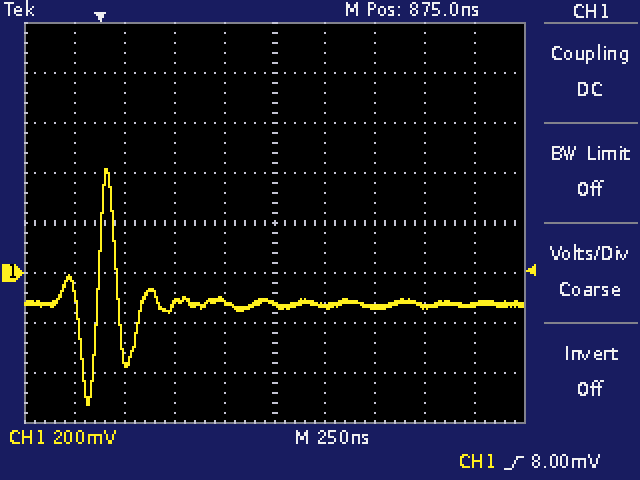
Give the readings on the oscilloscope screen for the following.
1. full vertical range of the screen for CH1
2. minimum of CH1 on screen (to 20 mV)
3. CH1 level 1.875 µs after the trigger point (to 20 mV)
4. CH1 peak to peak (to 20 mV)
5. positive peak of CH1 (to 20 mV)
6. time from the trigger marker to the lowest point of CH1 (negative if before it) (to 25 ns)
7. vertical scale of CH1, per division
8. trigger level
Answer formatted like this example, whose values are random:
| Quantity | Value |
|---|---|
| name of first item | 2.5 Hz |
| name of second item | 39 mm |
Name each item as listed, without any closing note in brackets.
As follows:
| Quantity | Value |
|---|---|
| full vertical range of the screen for CH1 | 1.6 V |
| minimum of CH1 on screen | -520 mV |
| CH1 level 1.875 µs after the trigger point | -120 mV |
| CH1 peak to peak | 940 mV |
| positive peak of CH1 | 420 mV |
| time from the trigger marker to the lowest point of CH1 (negative if before it) | -50 ns |
| vertical scale of CH1, per division | 200 mV |
| trigger level | 8.00 mV |
